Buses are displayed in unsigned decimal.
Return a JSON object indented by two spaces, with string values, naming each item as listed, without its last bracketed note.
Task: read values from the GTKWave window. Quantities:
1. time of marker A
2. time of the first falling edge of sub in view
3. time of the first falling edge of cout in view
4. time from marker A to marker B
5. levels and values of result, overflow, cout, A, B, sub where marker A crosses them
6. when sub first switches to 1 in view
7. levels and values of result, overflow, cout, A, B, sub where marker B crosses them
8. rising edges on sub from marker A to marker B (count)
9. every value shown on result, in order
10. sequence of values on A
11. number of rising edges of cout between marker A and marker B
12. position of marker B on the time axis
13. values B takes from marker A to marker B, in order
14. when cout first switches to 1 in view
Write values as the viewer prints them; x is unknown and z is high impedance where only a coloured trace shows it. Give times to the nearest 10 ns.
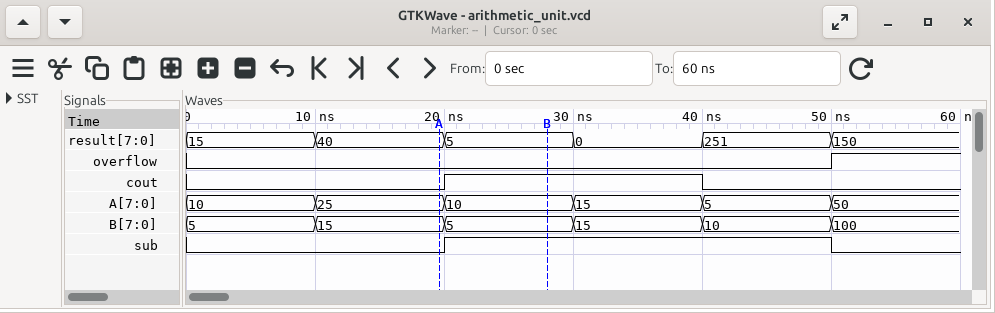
{
  "time of marker A": "20 ns",
  "time of the first falling edge of sub in view": "50 ns",
  "time of the first falling edge of cout in view": "40 ns",
  "time from marker A to marker B": "10 ns",
  "levels and values of result, overflow, cout, A, B, sub where marker A crosses them": "result=40, overflow=0, cout=0, A=25, B=15, sub=0",
  "when sub first switches to 1 in view": "20 ns",
  "levels and values of result, overflow, cout, A, B, sub where marker B crosses them": "result=5, overflow=0, cout=1, A=10, B=5, sub=1",
  "rising edges on sub from marker A to marker B": "1",
  "every value shown on result, in order": "15, 40, 5, 0, 251, 150",
  "sequence of values on A": "10, 25, 10, 15, 5, 50",
  "number of rising edges of cout between marker A and marker B": "1",
  "position of marker B on the time axis": "30 ns",
  "values B takes from marker A to marker B, in order": "15, 5",
  "when cout first switches to 1 in view": "20 ns"
}
